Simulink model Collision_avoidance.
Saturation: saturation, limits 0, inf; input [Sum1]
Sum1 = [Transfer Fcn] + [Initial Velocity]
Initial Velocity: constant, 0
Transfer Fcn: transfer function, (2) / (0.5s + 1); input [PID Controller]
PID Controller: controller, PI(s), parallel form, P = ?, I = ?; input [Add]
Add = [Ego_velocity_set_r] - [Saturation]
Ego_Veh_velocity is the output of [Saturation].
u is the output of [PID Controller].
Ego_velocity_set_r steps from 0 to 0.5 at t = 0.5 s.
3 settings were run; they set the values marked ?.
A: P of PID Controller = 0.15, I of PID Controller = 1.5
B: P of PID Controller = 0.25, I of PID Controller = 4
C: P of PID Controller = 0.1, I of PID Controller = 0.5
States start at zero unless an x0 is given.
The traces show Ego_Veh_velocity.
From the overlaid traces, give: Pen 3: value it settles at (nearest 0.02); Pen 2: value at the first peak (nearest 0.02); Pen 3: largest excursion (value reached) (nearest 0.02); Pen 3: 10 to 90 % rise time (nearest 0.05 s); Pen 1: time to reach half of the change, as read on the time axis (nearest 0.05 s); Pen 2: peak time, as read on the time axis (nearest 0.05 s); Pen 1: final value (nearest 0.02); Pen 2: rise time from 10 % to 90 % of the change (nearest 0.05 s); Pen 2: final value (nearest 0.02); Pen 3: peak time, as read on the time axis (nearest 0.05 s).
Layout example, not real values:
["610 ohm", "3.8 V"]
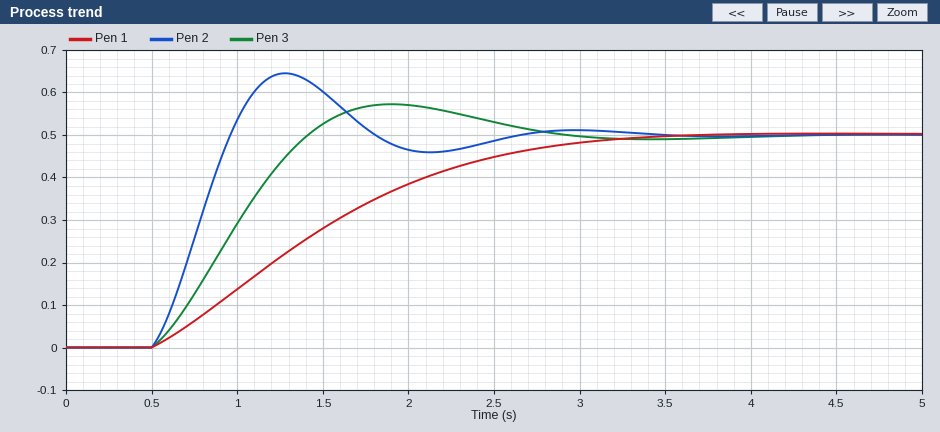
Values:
["0.50", "0.64", "0.58", "0.65 s", "1.40 s", "1.30 s", "0.50", "0.35 s", "0.50", "1.90 s"]
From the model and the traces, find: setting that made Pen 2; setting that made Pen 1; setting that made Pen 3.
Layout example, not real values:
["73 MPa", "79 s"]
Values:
["B", "C", "A"]
